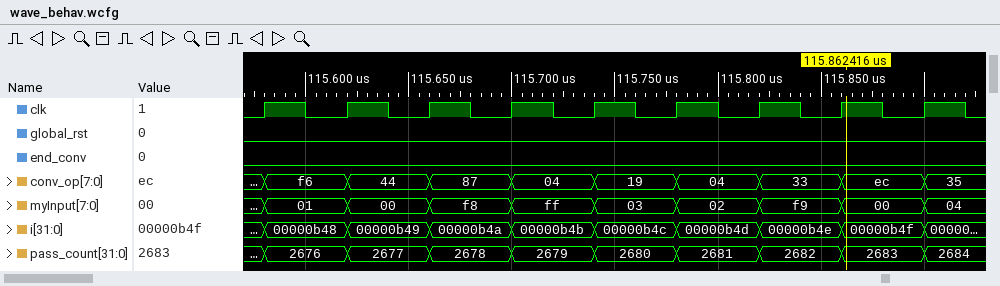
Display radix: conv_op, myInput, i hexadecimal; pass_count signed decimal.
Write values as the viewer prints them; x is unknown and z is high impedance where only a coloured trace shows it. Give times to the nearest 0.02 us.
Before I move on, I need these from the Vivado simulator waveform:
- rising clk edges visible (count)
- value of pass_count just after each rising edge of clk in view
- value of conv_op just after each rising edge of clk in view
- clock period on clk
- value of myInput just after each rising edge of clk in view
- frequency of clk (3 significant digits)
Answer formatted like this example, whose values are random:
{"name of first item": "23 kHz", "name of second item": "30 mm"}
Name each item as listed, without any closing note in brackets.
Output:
{"rising clk edges visible": "9", "value of pass_count just after each rising edge of clk in view": "2676, 2677, 2678, 2679, 2680, 2681, 2682, 2683, 2684", "value of conv_op just after each rising edge of clk in view": "f6, 44, 87, 04, 19, 04, 33, ec, 35", "clock period on clk": "0.04 us", "value of myInput just after each rising edge of clk in view": "01, 00, f8, ff, 03, 02, f9, 00, 04", "frequency of clk": "25.0 MHz"}
